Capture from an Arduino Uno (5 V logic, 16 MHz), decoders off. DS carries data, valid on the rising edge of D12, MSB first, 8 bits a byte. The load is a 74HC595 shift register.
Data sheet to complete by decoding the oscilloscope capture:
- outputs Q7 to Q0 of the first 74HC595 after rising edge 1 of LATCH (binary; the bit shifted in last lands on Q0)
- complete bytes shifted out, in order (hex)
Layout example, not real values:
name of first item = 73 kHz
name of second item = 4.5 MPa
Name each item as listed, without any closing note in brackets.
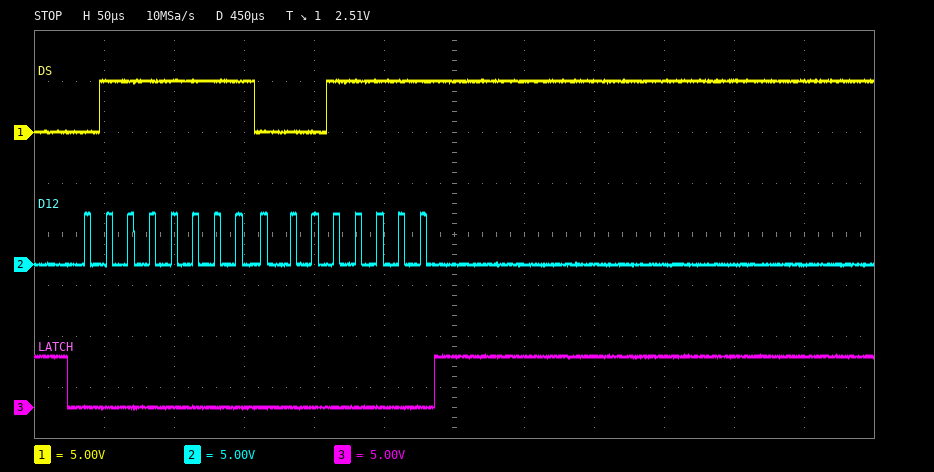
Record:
outputs Q7 to Q0 of the first 74HC595 after rising edge 1 of LATCH = 00011111
complete bytes shifted out, in order = 7F 1F
